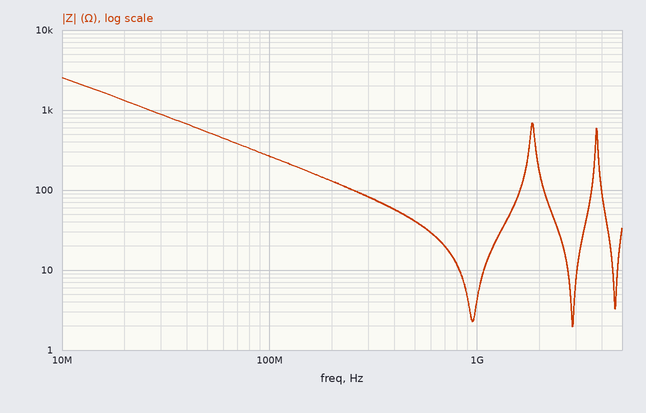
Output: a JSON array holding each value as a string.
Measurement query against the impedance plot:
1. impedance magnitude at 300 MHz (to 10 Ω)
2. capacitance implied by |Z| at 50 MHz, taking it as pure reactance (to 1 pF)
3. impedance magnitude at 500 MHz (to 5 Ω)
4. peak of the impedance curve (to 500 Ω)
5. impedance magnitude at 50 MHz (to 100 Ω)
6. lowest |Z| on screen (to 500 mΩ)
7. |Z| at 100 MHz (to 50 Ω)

["80 Ω", "6 pF", "40 Ω", "2.5 kΩ", "500 Ω", "2.0 Ω", "250 Ω"]
